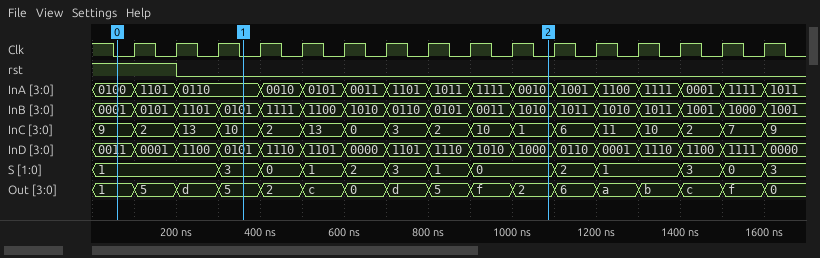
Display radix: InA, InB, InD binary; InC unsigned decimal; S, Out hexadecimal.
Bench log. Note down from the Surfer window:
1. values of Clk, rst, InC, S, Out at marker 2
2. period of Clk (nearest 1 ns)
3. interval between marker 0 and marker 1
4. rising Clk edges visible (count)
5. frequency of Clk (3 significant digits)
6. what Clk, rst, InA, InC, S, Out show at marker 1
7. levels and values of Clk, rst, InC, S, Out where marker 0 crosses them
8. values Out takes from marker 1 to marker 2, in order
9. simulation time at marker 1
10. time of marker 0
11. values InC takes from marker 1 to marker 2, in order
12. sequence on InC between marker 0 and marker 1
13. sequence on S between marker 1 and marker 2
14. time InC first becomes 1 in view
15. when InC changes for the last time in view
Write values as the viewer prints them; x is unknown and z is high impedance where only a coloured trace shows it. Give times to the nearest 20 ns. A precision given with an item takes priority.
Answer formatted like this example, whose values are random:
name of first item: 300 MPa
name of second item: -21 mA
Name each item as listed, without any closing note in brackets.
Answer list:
values of Clk, rst, InC, S, Out at marker 2: Clk=0, rst=0, InC=1, S=0, Out=2
period of Clk: 100 ns
interval between marker 0 and marker 1: 300 ns
rising Clk edges visible: 16
frequency of Clk: 10.0 MHz
what Clk, rst, InA, InC, S, Out show at marker 1: Clk=0, rst=0, InA=0110, InC=10, S=3, Out=5
levels and values of Clk, rst, InC, S, Out where marker 0 crosses them: Clk=0, rst=1, InC=9, S=1, Out=1
values Out takes from marker 1 to marker 2, in order: 5, 2, c, 0, d, 5, f, 2
simulation time at marker 1: 360 ns
time of marker 0: 60 ns
values InC takes from marker 1 to marker 2, in order: 10, 2, 13, 0, 3, 2, 10, 1
sequence on InC between marker 0 and marker 1: 9, 2, 13, 10
sequence on S between marker 1 and marker 2: 3, 0, 1, 2, 3, 1, 0
time InC first becomes 1 in view: 1000 ns
when InC changes for the last time in view: 1600 ns
